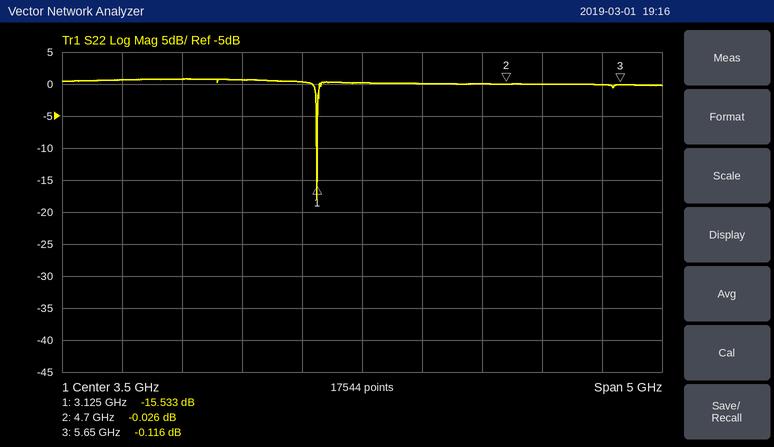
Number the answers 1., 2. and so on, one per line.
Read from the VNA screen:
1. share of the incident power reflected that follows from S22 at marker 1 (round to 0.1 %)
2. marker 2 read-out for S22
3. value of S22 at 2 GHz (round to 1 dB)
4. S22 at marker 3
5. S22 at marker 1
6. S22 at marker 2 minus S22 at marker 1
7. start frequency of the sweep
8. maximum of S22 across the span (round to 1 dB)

1. 2.8 %
2. -0.026 dB
3. 1 dB
4. -0.116 dB
5. -15.533 dB
6. 15.507 dB
7. 1 GHz
8. 1 dB
